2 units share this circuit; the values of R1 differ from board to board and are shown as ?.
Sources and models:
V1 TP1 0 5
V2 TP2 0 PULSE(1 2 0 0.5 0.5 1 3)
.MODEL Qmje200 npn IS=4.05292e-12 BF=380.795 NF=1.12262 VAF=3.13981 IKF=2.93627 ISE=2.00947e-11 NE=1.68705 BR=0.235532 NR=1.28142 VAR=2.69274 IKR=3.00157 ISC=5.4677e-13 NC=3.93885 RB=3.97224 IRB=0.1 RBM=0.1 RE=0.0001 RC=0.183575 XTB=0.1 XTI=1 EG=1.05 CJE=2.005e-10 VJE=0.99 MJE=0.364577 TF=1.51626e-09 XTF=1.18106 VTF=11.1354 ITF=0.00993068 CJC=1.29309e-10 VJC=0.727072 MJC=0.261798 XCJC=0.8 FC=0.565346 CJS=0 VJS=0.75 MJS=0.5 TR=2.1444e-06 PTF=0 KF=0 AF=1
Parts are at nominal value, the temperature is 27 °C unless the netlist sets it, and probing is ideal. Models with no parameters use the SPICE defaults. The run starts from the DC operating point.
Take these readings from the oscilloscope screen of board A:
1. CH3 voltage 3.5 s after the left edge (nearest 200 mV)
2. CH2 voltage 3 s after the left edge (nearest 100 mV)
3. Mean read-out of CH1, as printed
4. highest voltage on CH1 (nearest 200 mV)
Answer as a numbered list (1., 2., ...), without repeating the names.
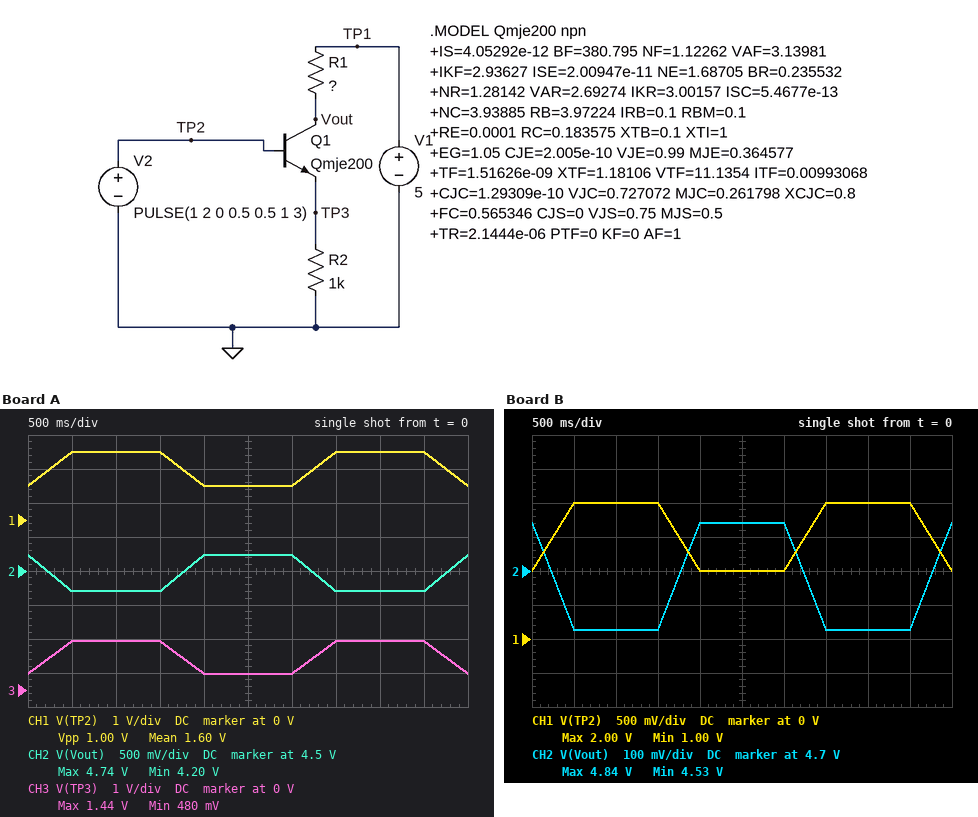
1. 1.4 V
2. 4.7 V
3. 1.60 V
4. 2.0 V
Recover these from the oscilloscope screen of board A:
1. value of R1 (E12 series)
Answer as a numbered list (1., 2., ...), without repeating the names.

1. 560 Ω
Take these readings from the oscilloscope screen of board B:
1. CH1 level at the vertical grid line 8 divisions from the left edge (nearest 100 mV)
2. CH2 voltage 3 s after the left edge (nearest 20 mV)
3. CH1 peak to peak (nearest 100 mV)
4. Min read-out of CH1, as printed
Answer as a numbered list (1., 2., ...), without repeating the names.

1. 2.0 V
2. 4.84 V
3. 1.0 V
4. 1.00 V
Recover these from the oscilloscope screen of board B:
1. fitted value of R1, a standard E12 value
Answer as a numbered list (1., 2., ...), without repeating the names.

1. 330 Ω
